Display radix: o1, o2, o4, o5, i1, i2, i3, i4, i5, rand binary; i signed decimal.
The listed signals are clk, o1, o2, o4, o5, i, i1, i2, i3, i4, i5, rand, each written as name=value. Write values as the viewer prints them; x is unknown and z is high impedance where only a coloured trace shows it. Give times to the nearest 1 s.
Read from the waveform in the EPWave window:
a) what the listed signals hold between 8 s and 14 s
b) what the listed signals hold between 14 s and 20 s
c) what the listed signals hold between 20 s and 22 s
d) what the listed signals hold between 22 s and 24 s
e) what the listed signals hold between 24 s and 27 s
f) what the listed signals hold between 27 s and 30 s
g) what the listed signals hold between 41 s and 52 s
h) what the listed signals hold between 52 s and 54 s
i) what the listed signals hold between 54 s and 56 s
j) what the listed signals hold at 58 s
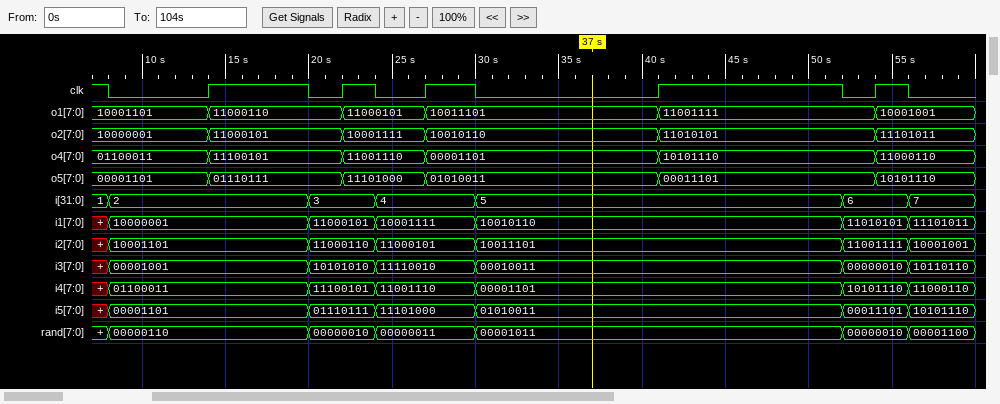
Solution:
clk=0, o1=10001101, o2=10000001, o4=01100011, o5=00001101, i=2, i1=10000001, i2=10001101, i3=00001001, i4=01100011, i5=00001101, rand=00000110
clk=1, o1=11000110, o2=11000101, o4=11100101, o5=01110111, i=2, i1=10000001, i2=10001101, i3=00001001, i4=01100011, i5=00001101, rand=00000110
clk=0, o1=11000110, o2=11000101, o4=11100101, o5=01110111, i=3, i1=11000101, i2=11000110, i3=10101010, i4=11100101, i5=01110111, rand=00000010
clk=1, o1=11000101, o2=10001111, o4=11001110, o5=11101000, i=3, i1=11000101, i2=11000110, i3=10101010, i4=11100101, i5=01110111, rand=00000010
clk=0, o1=11000101, o2=10001111, o4=11001110, o5=11101000, i=4, i1=10001111, i2=11000101, i3=11110010, i4=11001110, i5=11101000, rand=00000011
clk=1, o1=10011101, o2=10010110, o4=00001101, o5=01010011, i=4, i1=10001111, i2=11000101, i3=11110010, i4=11001110, i5=11101000, rand=00000011
clk=1, o1=11001111, o2=11010101, o4=10101110, o5=00011101, i=5, i1=10010110, i2=10011101, i3=00010011, i4=00001101, i5=01010011, rand=00001011
clk=0, o1=11001111, o2=11010101, o4=10101110, o5=00011101, i=6, i1=11010101, i2=11001111, i3=00000010, i4=10101110, i5=00011101, rand=00000010
clk=1, o1=10001001, o2=11101011, o4=11000110, o5=10101110, i=6, i1=11010101, i2=11001111, i3=00000010, i4=10101110, i5=00011101, rand=00000010
clk=0, o1=10001001, o2=11101011, o4=11000110, o5=10101110, i=7, i1=11101011, i2=10001001, i3=10110110, i4=11000110, i5=10101110, rand=00001100
